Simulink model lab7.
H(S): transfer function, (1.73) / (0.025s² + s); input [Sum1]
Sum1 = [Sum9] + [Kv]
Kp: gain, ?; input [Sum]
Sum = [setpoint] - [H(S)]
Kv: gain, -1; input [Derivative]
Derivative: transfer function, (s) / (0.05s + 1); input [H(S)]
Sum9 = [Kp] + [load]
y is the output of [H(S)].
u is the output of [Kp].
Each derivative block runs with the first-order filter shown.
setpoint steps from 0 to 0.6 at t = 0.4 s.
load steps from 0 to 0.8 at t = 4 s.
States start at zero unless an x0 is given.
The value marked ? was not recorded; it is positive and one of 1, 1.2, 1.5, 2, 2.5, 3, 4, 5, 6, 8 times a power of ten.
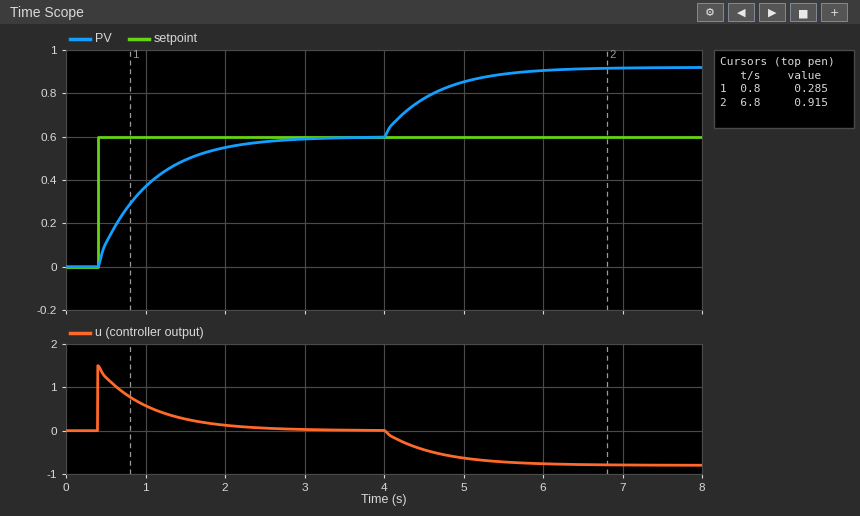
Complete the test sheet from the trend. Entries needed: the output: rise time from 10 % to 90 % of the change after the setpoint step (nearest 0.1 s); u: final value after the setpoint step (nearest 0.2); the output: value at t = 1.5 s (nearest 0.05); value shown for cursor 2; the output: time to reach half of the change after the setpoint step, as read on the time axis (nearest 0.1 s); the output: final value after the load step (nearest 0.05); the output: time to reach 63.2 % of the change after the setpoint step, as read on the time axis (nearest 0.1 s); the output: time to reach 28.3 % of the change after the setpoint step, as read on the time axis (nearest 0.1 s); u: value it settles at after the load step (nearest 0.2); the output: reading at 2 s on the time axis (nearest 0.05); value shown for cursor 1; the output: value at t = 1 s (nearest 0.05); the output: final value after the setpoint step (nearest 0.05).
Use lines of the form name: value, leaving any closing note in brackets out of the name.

the output: rise time from 10 % to 90 % of the change after the setpoint step: 1.4 s
u: final value after the setpoint step: 0.0
the output: value at t = 1.5 s: 0.50
value shown for cursor 2: 0.915
the output: time to reach half of the change after the setpoint step, as read on the time axis: 0.8 s
the output: final value after the load step: 0.90
the output: time to reach 63.2 % of the change after the setpoint step, as read on the time axis: 1.0 s
the output: time to reach 28.3 % of the change after the setpoint step, as read on the time axis: 0.6 s
u: value it settles at after the load step: -0.8
the output: reading at 2 s on the time axis: 0.55
value shown for cursor 1: 0.285
the output: value at t = 1 s: 0.35
the output: final value after the setpoint step: 0.60
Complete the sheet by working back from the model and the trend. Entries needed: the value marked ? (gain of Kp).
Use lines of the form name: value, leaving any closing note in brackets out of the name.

the value marked ?: 2.5
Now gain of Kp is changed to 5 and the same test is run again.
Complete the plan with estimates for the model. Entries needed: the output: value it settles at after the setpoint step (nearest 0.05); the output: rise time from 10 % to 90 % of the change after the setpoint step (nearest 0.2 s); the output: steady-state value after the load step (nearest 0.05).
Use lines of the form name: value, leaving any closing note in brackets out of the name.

the output: value it settles at after the setpoint step: 0.60
the output: rise time from 10 % to 90 % of the change after the setpoint step: 0.8 s
the output: steady-state value after the load step: 0.75
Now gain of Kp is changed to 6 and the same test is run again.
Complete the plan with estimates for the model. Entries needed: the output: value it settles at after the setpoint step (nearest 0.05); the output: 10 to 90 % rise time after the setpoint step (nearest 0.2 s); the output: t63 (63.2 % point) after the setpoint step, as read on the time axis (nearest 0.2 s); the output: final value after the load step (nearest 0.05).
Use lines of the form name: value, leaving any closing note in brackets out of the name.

the output: value it settles at after the setpoint step: 0.60
the output: 10 to 90 % rise time after the setpoint step: 0.6 s
the output: t63 (63.2 % point) after the setpoint step, as read on the time axis: 0.6 s
the output: final value after the load step: 0.75
